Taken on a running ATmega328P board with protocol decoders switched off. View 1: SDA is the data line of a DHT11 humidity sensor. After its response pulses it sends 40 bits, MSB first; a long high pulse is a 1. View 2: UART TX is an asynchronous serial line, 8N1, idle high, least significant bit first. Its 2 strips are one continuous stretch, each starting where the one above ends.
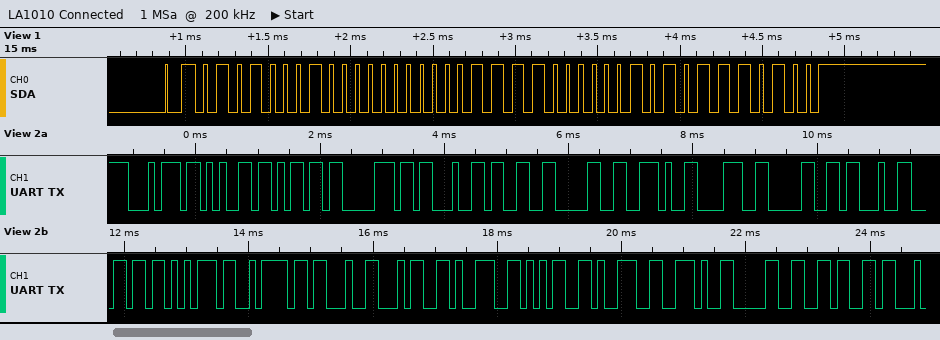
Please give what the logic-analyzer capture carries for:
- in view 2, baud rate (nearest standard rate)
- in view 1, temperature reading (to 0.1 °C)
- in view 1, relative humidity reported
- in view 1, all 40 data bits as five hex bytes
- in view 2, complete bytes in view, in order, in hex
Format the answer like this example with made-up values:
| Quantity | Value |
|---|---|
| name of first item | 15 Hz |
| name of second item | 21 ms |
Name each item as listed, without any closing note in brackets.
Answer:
| Quantity | Value |
|---|---|
| in view 2, baud rate | 9600 baud |
| in view 1, temperature reading | 30.5 °C |
| in view 1, relative humidity reported | 81 % |
| in view 1, all 40 data bits as five hex bytes | 51 00 1E 05 74 |
| in view 2, complete bytes in view, in order, in hex | 74 65 6D 70 23 33 30 2E 38 30 23 6C 75 7A 23 34 39 35 39 2E 30 36 |
